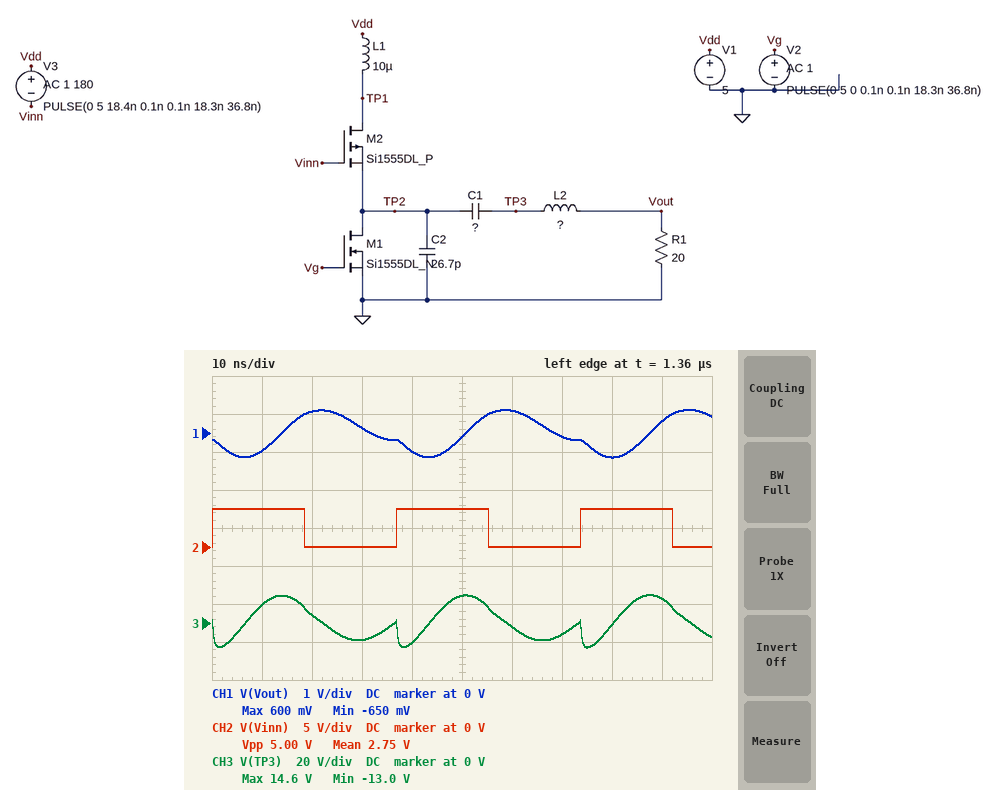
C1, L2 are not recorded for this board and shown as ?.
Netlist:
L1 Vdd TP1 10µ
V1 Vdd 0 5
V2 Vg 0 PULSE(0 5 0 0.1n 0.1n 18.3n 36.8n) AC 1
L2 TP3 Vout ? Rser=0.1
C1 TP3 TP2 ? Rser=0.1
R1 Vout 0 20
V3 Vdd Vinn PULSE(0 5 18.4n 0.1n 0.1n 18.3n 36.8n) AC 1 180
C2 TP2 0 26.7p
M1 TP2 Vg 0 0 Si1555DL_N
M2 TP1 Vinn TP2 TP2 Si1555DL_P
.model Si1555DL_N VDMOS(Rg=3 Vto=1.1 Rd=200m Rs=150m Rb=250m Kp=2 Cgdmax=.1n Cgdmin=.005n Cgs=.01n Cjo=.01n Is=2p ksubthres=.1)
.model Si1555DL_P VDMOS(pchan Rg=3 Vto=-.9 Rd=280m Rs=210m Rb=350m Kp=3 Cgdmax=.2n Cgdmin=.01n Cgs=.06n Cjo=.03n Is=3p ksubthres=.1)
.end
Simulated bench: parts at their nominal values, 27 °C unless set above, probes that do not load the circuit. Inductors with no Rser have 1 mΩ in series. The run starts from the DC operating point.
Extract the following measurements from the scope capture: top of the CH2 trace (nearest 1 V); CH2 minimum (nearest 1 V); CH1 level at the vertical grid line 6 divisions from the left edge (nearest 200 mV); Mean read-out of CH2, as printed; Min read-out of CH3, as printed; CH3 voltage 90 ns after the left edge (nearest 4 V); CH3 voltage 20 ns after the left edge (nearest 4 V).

5 V
0 V
600 mV
2.75 V
-13.0 V
12 V
4 V
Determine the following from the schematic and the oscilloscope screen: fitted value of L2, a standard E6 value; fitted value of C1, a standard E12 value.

2.2 µH
10 pF
